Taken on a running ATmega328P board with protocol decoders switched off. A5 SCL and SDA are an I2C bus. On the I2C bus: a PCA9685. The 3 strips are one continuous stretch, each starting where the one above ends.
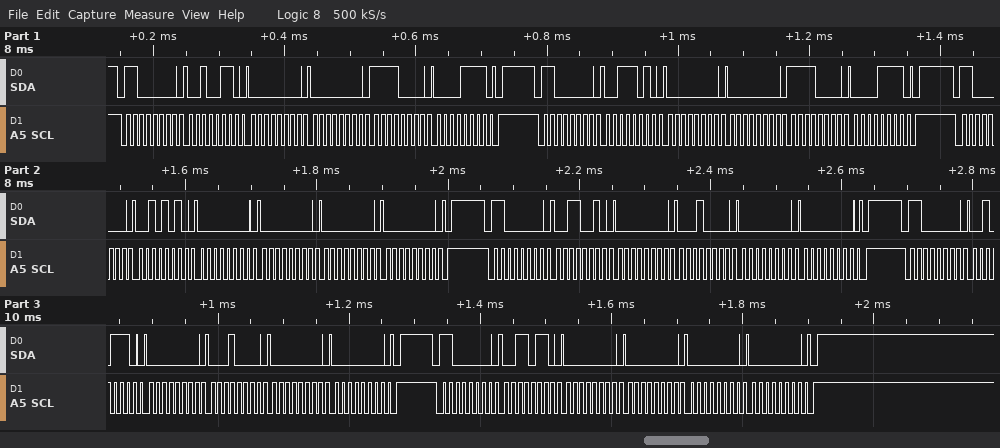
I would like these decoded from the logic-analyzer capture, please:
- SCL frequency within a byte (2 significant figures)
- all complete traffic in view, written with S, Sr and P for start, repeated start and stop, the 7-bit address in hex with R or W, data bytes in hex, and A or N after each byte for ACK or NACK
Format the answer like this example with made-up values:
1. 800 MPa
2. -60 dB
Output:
1. 100 kHz
2. S 60W A 26 A 00 A 00 A F0 A 0F A P S 60W A 3A A 00 A 00 A F0 A 0F A P S 60W A 2A A 00 A 00 A 00 A 00 A P S 60W A 32 A 00 A 10 A 00 A 00 A P S 60W A 2E A 00 A 10 A 00 A 00 A P S 60W A 36 A 00 A 00 A 00 A 00 A P
